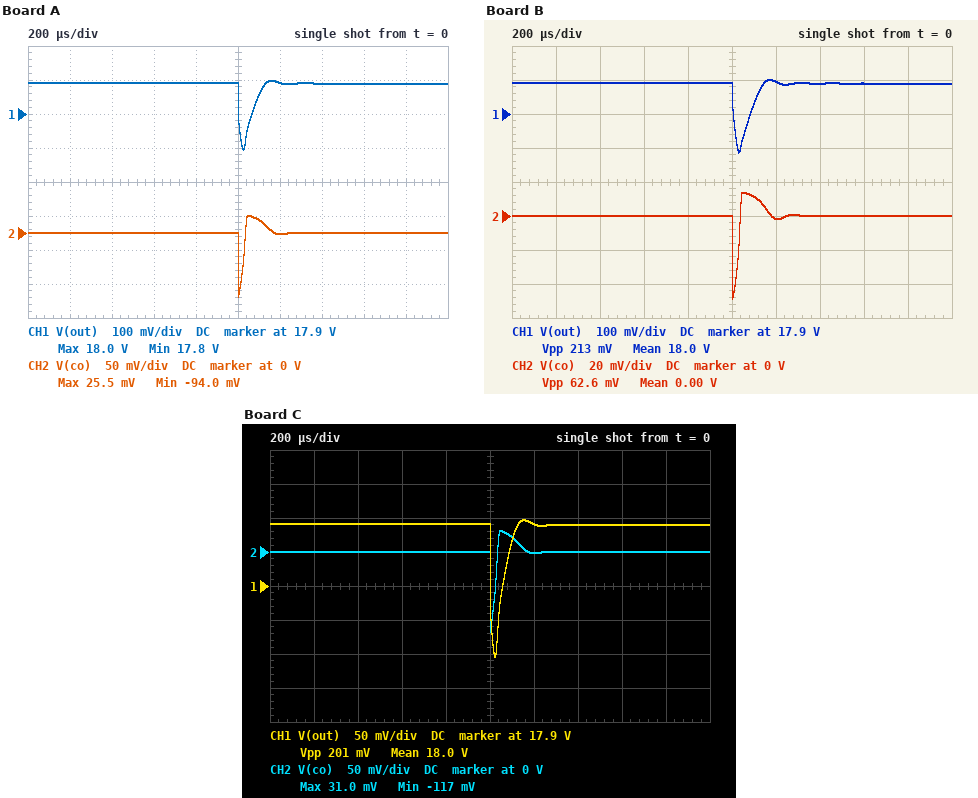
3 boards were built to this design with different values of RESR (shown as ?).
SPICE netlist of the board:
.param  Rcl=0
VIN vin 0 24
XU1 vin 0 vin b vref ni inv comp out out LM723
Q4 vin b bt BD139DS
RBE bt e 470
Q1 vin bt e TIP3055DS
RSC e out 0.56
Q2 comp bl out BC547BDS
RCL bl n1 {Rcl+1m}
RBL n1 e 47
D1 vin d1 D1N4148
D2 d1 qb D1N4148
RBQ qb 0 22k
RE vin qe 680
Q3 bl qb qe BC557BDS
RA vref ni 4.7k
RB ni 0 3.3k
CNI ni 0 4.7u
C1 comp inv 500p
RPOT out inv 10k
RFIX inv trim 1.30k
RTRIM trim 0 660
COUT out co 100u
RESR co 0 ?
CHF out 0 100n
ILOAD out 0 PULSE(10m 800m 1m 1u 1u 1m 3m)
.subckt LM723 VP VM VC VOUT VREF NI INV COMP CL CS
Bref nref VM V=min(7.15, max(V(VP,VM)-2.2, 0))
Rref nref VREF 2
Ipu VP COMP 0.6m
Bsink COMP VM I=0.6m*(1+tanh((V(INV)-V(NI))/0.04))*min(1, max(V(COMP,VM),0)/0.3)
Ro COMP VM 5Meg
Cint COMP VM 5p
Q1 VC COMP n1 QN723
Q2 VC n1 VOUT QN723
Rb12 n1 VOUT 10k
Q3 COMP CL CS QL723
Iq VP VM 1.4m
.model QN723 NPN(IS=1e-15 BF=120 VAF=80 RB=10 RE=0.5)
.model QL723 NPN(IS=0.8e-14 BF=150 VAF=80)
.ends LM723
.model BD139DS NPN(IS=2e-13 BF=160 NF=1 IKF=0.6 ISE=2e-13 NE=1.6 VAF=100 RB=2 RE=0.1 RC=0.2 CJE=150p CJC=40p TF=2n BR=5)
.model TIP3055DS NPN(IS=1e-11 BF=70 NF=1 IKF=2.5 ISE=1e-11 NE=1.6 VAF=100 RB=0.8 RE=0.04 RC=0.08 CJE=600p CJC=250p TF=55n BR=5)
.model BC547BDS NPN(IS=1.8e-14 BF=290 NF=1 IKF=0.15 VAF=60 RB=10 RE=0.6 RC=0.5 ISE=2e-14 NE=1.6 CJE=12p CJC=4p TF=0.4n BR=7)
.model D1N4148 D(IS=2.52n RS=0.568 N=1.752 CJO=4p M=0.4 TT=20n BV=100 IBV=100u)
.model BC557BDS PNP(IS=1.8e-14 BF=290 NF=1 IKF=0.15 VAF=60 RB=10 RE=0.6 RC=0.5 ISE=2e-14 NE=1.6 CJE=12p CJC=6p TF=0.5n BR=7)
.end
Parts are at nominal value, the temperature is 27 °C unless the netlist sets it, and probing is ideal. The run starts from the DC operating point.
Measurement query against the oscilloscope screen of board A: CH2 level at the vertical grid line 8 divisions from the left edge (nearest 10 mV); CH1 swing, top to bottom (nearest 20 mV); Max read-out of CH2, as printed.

0 V
200 mV
25.5 mV
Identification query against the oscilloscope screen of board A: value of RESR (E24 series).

0.12 Ω
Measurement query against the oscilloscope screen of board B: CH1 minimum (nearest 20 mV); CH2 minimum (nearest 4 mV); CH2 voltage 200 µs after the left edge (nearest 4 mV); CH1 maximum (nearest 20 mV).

17.78 V
-48 mV
0 V
18.00 V
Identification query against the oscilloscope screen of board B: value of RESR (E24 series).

0.062 Ω
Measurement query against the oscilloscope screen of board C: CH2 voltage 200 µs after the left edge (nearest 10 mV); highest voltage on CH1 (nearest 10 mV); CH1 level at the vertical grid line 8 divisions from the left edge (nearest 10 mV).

0 V
18.00 V
17.99 V
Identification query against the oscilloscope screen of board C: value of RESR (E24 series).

0.15 Ω
